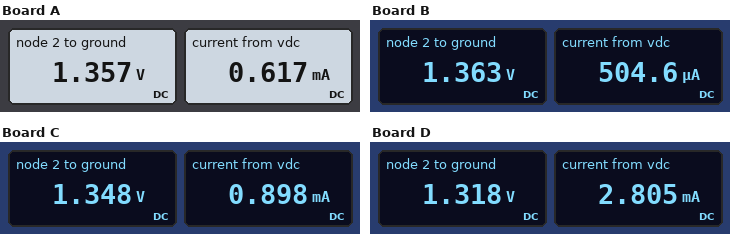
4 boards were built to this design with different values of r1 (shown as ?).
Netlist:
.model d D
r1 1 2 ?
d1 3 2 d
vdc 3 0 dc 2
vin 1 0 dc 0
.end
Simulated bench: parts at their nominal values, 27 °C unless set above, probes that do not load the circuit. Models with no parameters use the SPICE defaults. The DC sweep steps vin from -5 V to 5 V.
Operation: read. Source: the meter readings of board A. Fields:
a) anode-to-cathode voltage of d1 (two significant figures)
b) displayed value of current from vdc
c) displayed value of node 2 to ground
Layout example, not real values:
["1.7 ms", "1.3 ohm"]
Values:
["640 mV", "0.617 mA", "1.357 V"]
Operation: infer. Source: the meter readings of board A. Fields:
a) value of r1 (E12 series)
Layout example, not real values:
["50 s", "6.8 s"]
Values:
["2.2 kΩ"]
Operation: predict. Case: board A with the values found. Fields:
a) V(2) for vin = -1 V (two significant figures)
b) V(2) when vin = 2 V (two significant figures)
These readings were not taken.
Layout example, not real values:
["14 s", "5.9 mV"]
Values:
["1.3 V", "2.0 V"]
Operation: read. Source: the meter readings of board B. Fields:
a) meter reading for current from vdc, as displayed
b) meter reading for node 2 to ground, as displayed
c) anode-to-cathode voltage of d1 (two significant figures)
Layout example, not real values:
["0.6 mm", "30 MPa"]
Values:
["504.6 µA", "1.363 V", "640 mV"]
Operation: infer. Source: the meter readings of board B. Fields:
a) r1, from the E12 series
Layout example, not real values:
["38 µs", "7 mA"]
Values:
["2.7 kΩ"]
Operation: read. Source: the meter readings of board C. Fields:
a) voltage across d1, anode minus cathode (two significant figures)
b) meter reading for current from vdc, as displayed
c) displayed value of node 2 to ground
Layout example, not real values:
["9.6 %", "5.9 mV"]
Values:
["650 mV", "0.898 mA", "1.348 V"]
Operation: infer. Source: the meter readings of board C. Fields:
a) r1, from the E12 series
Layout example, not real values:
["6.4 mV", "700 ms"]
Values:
["1.5 kΩ"]
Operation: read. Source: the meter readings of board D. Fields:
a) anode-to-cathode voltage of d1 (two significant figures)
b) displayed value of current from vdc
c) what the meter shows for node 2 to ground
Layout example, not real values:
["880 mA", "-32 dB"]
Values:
["680 mV", "2.805 mA", "1.318 V"]
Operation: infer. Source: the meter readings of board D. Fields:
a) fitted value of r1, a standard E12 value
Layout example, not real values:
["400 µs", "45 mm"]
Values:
["470 Ω"]
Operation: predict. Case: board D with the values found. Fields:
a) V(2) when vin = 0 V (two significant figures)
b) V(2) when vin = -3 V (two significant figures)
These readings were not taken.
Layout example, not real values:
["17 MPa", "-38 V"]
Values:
["1.3 V", "1.3 V"]
